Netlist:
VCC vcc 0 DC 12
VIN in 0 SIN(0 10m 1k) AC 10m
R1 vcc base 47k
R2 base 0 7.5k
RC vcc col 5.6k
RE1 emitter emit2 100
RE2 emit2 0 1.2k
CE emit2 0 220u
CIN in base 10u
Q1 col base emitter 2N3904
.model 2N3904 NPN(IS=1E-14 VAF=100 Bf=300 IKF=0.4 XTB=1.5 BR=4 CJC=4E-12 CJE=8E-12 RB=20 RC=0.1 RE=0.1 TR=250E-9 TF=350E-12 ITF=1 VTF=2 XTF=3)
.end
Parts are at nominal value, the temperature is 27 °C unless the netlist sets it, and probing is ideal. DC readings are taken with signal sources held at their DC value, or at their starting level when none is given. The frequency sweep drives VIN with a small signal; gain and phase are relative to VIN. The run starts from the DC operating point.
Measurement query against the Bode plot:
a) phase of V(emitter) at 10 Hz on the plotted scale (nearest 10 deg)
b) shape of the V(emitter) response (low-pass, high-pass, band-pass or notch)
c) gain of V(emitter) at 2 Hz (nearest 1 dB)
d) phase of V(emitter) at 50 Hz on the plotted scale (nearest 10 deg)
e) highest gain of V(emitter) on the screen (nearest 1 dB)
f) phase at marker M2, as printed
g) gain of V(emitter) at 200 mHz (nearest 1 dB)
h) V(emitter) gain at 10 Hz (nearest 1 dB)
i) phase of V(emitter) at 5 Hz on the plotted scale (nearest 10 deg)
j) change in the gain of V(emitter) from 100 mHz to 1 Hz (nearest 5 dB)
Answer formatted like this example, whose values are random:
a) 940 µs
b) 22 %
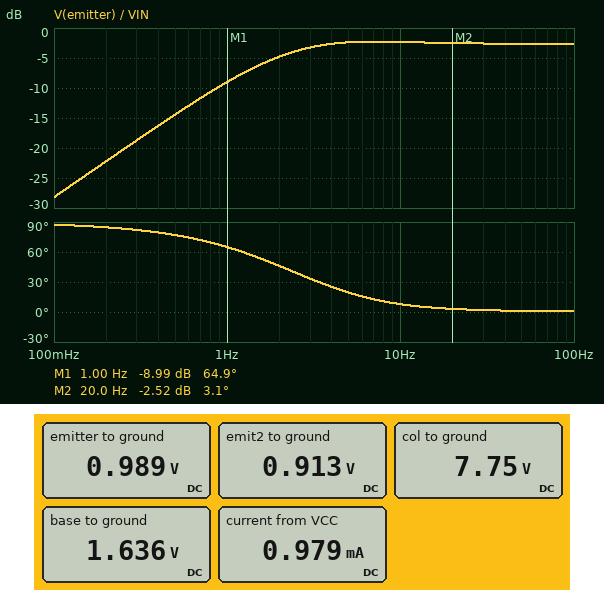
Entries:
a) 10 deg
b) high-pass
c) -5 dB
d) 0 deg
e) -2 dB
f) 3.1 deg
g) -22 dB
h) -2 dB
i) 20 deg
j) 20 dB
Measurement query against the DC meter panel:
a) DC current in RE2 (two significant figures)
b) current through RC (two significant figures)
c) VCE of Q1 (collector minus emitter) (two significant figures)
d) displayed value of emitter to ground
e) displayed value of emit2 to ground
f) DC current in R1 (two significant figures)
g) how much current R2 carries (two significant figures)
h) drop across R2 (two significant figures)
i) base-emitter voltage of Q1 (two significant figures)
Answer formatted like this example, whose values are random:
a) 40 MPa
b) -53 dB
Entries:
a) 760 µA
b) 760 µA
c) 6.8 V
d) 0.989 V
e) 0.913 V
f) 220 µA
g) 220 µA
h) 1.6 V
i) 650 mV
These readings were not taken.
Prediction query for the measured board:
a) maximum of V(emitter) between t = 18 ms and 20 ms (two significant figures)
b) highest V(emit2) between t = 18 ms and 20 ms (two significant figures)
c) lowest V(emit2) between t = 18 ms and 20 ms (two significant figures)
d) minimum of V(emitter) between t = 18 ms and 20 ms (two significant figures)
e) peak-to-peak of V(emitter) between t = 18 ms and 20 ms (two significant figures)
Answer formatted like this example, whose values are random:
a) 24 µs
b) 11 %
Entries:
a) 1.0 V
b) 910 mV
c) 910 mV
d) 980 mV
e) 15 mV
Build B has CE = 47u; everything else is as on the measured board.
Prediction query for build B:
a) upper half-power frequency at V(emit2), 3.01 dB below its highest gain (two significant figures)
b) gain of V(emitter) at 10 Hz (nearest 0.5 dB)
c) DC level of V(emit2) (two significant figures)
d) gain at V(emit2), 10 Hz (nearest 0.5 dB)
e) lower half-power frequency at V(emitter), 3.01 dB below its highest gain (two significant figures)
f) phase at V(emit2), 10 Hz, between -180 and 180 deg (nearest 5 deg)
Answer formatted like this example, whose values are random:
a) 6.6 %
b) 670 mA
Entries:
a) 33 Hz
b) -1.0 dB
c) 910 mV
d) -2.0 dB
e) 2.2 Hz
f) -5 deg
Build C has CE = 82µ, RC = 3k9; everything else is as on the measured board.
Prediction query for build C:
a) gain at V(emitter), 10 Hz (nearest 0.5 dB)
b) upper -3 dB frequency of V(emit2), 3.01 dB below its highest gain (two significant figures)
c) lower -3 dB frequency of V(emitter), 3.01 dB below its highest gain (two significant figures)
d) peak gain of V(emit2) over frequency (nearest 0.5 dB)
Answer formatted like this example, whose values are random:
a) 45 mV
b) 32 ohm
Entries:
a) -1.0 dB
b) 21 Hz
c) 2.1 Hz
d) -2.5 dB
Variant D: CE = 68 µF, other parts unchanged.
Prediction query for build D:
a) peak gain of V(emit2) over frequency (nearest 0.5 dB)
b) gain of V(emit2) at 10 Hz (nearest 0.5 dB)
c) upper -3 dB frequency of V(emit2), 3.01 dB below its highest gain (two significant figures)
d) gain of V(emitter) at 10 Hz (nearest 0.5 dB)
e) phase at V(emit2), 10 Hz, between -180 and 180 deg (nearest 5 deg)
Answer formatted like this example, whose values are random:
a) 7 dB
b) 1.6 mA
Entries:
a) -2.0 dB
b) -2.5 dB
c) 24 Hz
d) -1.0 dB
e) -15 deg
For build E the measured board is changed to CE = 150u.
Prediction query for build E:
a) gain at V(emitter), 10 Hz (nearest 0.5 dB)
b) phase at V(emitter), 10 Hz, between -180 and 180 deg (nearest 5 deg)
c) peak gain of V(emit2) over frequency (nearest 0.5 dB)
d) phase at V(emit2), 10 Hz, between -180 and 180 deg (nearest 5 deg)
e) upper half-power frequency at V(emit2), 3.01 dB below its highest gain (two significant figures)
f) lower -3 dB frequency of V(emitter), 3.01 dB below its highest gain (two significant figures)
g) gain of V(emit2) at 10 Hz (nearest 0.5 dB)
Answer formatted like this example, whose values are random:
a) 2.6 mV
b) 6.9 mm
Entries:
a) -2.0 dB
b) 5 deg
c) -3.5 dB
d) -35 deg
e) 13 Hz
f) 1.9 Hz
g) -5.0 dB
